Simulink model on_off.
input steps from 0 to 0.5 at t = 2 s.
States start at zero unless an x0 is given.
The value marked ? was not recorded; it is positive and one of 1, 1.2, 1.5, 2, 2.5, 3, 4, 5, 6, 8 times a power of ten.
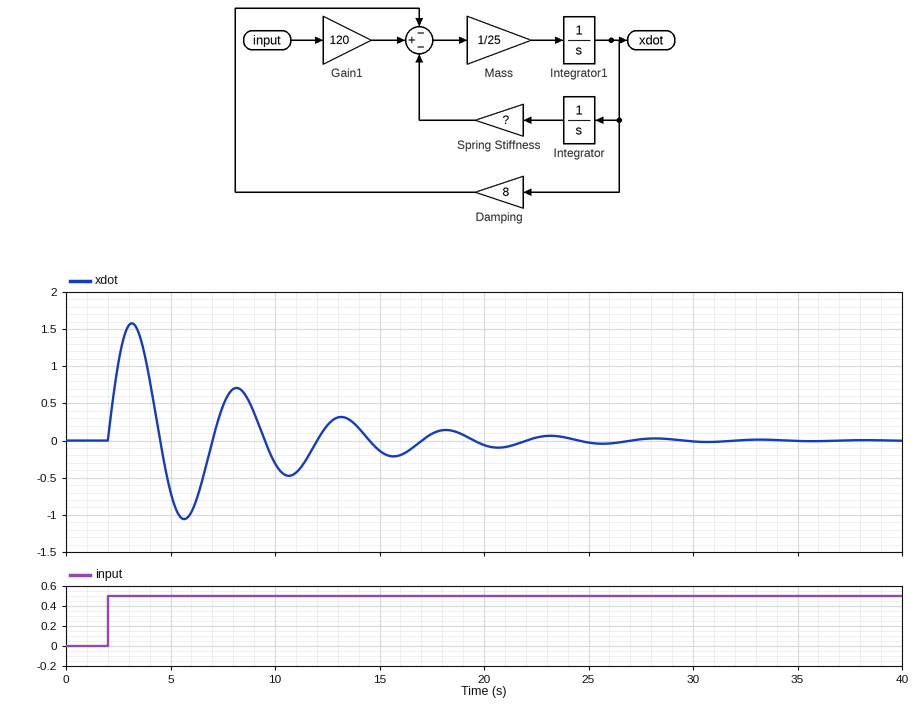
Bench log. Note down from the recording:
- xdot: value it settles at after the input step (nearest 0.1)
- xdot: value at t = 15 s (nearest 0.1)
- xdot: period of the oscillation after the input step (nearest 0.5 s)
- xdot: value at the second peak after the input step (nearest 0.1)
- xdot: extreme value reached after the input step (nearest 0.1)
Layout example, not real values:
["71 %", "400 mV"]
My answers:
["0.0", "-0.1", "5.0 s", "0.7", "1.6"]
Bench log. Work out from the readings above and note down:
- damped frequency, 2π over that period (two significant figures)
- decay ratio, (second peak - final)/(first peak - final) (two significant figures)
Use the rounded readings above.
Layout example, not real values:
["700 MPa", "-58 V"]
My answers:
["1.3 rad/s", "0.44"]
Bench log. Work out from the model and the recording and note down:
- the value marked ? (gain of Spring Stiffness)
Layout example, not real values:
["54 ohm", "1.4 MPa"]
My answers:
["40"]
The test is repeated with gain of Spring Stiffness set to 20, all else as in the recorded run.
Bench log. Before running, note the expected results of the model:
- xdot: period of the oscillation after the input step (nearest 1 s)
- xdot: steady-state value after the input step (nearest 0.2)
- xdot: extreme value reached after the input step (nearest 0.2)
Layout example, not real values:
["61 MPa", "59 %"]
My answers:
["7 s", "0.0", "2.0"]
